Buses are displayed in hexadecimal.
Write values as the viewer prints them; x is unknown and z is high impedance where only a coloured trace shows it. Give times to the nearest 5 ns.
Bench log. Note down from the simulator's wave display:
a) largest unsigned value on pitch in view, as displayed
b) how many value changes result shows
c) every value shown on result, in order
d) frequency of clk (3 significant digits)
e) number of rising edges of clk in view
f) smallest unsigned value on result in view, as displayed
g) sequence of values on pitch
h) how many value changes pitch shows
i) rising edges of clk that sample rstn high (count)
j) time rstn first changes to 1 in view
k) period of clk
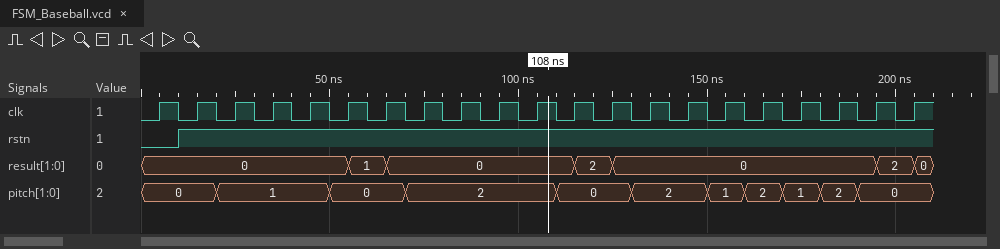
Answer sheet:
2
6
0, 1, 0, 2, 0, 2, 0
100 MHz
21
0
0, 1, 0, 2, 0, 2, 1, 2, 1, 2, 0
10
20
10 ns
10 ns
